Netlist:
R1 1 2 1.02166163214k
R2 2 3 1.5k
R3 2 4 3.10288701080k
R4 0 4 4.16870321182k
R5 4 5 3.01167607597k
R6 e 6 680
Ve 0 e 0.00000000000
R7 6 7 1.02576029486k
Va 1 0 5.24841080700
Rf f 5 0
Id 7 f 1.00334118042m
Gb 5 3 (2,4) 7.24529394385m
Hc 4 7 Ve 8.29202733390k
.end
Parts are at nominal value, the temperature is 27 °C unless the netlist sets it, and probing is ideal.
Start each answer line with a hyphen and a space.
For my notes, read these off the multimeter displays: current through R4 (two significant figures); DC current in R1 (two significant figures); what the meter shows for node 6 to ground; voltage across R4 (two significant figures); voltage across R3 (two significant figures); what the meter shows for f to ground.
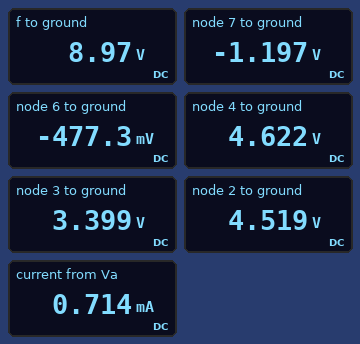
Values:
- 1.1 mA
- 710 µA
- -477.3 mV
- 4.6 V
- 100 mV
- 8.97 V
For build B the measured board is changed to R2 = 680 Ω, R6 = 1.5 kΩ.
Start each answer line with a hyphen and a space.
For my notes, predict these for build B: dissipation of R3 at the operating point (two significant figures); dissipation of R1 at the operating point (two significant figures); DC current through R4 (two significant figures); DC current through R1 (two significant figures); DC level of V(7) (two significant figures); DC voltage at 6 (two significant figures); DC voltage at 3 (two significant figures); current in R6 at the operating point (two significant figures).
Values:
- 2.5 µW
- 380 µW
- 1.1 mA
- 610 µA
- -2.1 V
- -1.2 V
- 4.2 V
- 820 µA
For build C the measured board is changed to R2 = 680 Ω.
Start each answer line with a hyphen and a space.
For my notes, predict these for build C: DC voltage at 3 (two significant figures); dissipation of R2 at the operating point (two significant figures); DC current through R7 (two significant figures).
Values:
- 4.0 V
- 380 µW
- 700 µA
